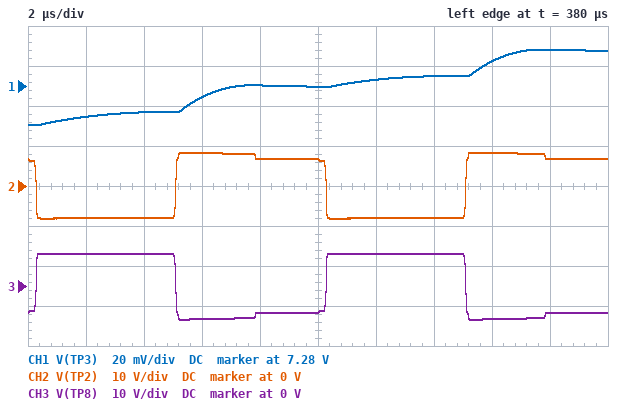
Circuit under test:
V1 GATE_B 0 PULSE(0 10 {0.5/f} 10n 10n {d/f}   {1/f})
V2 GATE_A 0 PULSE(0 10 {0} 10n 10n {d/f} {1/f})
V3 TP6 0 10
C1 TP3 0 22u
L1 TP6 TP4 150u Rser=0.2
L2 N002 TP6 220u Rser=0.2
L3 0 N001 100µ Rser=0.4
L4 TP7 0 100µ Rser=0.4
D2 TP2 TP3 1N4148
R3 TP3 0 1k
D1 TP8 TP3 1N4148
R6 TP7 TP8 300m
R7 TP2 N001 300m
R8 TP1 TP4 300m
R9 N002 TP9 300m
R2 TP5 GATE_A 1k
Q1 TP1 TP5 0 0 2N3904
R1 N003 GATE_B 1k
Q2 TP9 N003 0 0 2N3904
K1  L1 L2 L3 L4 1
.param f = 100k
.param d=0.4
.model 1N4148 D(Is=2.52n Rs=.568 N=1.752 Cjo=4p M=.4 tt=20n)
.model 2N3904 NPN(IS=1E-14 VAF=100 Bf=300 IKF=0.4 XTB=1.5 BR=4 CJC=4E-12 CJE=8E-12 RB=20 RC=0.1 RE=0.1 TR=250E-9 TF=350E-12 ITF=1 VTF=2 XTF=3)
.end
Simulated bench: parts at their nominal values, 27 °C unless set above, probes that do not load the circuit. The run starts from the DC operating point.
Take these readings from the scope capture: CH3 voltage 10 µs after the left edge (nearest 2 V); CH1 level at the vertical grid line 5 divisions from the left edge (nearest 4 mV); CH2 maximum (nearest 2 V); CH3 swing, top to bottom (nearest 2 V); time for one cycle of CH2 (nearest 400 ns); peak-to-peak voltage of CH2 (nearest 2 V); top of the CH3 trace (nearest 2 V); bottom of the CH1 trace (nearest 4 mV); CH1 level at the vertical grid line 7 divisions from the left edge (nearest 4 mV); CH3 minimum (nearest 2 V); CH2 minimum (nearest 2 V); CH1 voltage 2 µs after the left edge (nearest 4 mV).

-6 V
7.280 V
8 V
16 V
10.0 µs
16 V
8 V
7.260 V
7.284 V
-8 V
-8 V
7.264 V
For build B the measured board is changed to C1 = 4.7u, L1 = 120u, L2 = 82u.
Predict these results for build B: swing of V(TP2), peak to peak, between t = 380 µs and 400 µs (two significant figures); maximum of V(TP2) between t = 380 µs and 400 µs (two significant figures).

26 V
13 V
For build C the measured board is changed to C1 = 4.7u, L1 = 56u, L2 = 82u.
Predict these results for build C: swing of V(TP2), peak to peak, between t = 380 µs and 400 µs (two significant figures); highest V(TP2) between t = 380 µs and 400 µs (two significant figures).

32 V
16 V
